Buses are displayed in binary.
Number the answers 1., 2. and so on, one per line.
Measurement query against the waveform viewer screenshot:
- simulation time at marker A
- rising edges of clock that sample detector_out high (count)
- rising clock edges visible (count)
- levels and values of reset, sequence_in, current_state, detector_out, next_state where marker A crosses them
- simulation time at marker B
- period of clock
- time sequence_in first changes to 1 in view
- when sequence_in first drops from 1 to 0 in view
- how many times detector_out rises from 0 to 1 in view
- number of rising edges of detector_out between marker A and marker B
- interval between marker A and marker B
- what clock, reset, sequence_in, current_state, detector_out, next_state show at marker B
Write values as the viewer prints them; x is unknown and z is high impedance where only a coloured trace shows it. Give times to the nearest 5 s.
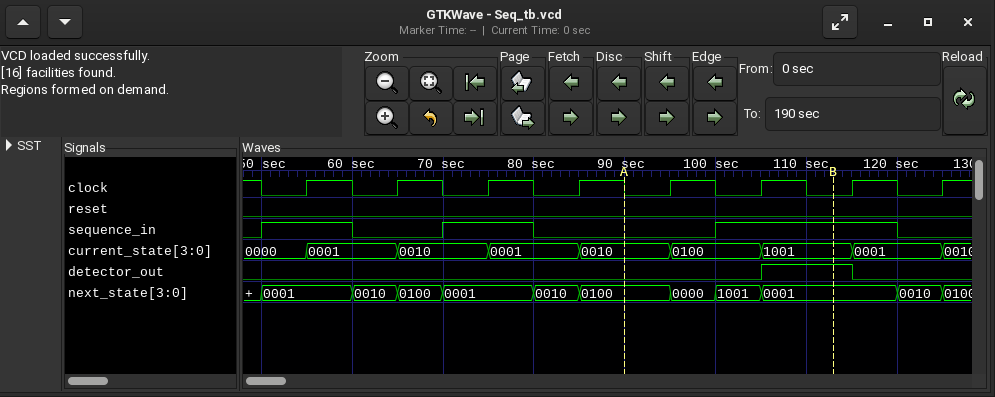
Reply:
1. 90 s
2. 1
3. 8
4. reset=0, sequence_in=0, current_state=0010, detector_out=0, next_state=0100
5. 115 s
6. 10 s
7. 50 s
8. 60 s
9. 1
10. 1
11. 25 s
12. clock=0, reset=0, sequence_in=1, current_state=1001, detector_out=1, next_state=0001
